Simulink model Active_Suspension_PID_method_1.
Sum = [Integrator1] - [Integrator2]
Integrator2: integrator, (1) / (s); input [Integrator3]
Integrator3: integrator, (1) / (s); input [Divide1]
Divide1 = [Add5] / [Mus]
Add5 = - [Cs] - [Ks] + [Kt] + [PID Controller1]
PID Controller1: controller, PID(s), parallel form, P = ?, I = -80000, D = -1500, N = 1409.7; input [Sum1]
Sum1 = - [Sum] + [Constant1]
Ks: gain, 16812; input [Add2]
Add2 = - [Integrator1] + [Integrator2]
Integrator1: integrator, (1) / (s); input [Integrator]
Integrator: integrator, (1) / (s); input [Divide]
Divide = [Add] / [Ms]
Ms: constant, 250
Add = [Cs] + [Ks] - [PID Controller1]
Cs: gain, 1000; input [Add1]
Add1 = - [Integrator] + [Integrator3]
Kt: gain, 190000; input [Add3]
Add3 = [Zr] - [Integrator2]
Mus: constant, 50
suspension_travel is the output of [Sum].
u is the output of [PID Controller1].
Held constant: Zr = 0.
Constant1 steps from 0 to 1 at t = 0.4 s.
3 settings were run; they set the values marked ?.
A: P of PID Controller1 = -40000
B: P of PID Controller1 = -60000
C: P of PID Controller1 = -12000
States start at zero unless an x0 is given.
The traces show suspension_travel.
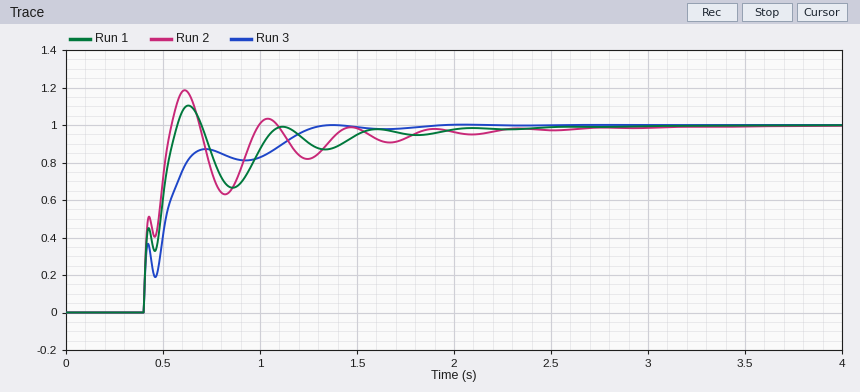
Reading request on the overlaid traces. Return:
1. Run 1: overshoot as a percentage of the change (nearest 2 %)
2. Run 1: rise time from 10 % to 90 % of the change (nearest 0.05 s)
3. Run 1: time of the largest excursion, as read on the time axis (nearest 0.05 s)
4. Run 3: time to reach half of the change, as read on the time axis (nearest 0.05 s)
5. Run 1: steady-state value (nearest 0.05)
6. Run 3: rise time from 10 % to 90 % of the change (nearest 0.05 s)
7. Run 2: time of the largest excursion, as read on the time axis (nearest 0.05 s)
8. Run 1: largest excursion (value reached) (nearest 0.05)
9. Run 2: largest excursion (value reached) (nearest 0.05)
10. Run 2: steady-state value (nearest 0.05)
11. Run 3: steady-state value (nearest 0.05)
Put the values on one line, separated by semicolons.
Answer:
10 %; 0.15 s; 0.65 s; 0.50 s; 1.00; 0.70 s; 0.60 s; 1.10; 1.20; 1.00; 1.00
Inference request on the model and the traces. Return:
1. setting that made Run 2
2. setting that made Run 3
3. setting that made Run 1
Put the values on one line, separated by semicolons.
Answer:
B; C; A
